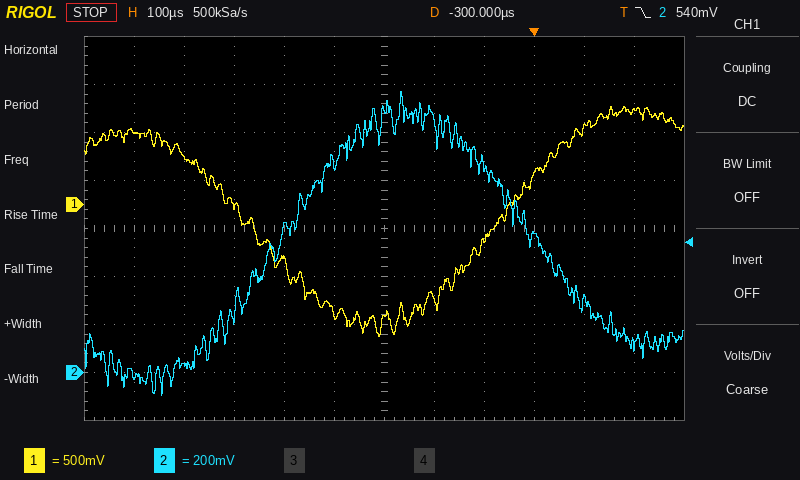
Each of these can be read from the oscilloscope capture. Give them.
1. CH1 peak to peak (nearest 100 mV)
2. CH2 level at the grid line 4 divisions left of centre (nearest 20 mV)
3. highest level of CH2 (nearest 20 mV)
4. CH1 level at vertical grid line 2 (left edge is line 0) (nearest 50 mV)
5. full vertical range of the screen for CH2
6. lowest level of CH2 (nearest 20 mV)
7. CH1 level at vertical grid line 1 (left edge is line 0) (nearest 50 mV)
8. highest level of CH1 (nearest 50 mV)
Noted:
2.40 V
20 mV
1.18 V
500 mV
1.6 V
-100 mV
750 mV
1.00 V
